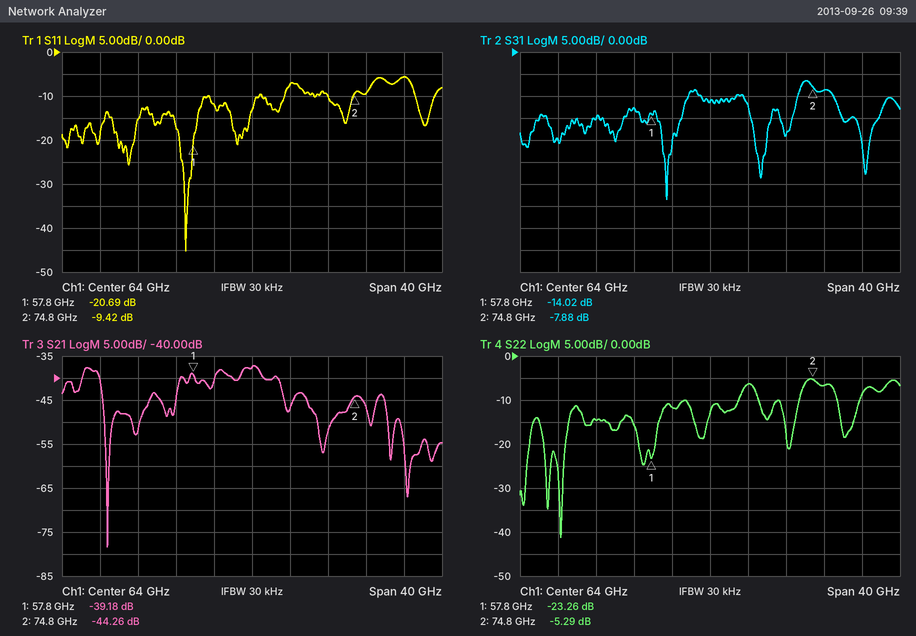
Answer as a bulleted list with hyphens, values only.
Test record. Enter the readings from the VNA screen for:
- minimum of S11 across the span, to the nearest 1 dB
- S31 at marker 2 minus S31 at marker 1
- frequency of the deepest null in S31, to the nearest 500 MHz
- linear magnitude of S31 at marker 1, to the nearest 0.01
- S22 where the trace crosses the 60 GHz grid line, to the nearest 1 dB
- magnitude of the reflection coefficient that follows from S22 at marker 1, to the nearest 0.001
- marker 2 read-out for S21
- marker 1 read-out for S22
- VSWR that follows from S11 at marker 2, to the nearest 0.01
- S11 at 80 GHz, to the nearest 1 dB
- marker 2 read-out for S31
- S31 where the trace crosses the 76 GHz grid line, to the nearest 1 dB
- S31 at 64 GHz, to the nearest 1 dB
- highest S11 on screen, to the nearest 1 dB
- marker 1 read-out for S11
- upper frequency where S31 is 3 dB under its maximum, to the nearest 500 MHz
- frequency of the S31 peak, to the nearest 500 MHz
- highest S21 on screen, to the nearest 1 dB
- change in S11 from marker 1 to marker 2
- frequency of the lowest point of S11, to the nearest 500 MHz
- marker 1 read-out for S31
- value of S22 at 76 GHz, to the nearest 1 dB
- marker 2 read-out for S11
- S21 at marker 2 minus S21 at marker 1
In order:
- -45 dB
- 6.14 dB
- 59.5 GHz
- 0.20
- -12 dB
- 0.069
- -44.26 dB
- -23.26 dB
- 2.02
- -6 dB
- -7.88 dB
- -9 dB
- -11 dB
- -6 dB
- -20.69 dB
- 77.0 GHz
- 74.0 GHz
- -37 dB
- 11.27 dB
- 57.0 GHz
- -14.02 dB
- -7 dB
- -9.42 dB
- -5.08 dB
